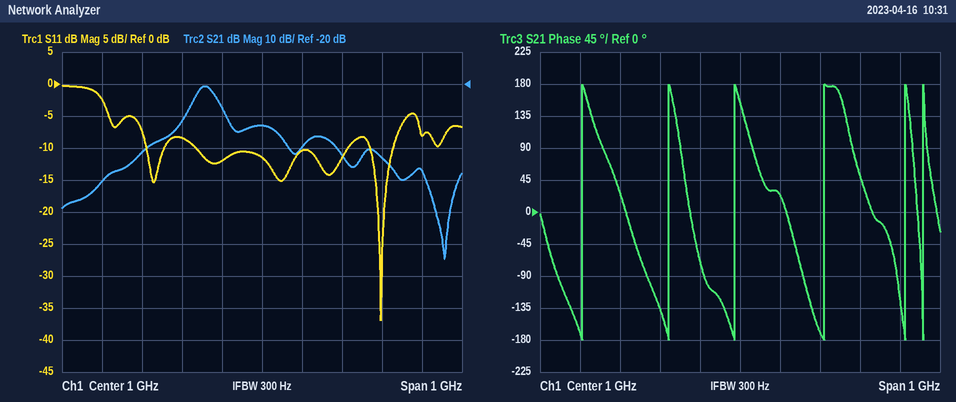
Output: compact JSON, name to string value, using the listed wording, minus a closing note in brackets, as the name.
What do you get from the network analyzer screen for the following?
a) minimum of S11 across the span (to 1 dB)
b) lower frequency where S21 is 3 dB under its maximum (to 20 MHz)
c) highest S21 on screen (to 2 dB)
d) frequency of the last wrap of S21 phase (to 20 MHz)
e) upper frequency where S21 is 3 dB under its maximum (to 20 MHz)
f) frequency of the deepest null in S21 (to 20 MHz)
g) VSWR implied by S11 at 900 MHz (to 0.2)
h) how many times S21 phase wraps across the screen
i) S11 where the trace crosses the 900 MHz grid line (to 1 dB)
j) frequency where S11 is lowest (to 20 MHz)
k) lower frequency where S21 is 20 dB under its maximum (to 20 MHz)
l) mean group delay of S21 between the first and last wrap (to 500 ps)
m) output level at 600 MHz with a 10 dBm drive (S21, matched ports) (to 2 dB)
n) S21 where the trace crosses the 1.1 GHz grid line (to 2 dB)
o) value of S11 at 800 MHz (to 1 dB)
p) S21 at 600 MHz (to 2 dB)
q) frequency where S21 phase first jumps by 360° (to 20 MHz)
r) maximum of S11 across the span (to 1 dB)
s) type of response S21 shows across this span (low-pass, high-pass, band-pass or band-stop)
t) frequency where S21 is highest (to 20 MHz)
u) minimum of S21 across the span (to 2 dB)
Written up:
{"minimum of S11 across the span": "-37 dB", "lower frequency where S21 is 3 dB under its maximum": "840 MHz", "highest S21 on screen": "-20 dB", "frequency of the last wrap of S21 phase": "1.46 GHz", "upper frequency where S21 is 3 dB under its maximum": "880 MHz", "frequency of the deepest null in S21": "1.46 GHz", "VSWR implied by S11 at 900 MHz": "1.6", "how many times S21 phase wraps across the screen": "6", "S11 where the trace crosses the 900 MHz grid line": "-12 dB", "frequency where S11 is lowest": "1.30 GHz", "lower frequency where S21 is 20 dB under its maximum": "700 MHz", "mean group delay of S21 between the first and last wrap": "6.0 ns", "output level at 600 MHz with a 10 dBm drive (S21, matched ports)": "-40 dBm", "S21 where the trace crosses the 1.1 GHz grid line": "-40 dB", "value of S11 at 800 MHz": "-8 dB", "S21 at 600 MHz": "-50 dB", "frequency where S21 phase first jumps by 360°": "600 MHz", "maximum of S11 across the span": "0 dB", "type of response S21 shows across this span": "band-pass", "frequency where S21 is highest": "860 MHz", "minimum of S21 across the span": "-74 dB"}
